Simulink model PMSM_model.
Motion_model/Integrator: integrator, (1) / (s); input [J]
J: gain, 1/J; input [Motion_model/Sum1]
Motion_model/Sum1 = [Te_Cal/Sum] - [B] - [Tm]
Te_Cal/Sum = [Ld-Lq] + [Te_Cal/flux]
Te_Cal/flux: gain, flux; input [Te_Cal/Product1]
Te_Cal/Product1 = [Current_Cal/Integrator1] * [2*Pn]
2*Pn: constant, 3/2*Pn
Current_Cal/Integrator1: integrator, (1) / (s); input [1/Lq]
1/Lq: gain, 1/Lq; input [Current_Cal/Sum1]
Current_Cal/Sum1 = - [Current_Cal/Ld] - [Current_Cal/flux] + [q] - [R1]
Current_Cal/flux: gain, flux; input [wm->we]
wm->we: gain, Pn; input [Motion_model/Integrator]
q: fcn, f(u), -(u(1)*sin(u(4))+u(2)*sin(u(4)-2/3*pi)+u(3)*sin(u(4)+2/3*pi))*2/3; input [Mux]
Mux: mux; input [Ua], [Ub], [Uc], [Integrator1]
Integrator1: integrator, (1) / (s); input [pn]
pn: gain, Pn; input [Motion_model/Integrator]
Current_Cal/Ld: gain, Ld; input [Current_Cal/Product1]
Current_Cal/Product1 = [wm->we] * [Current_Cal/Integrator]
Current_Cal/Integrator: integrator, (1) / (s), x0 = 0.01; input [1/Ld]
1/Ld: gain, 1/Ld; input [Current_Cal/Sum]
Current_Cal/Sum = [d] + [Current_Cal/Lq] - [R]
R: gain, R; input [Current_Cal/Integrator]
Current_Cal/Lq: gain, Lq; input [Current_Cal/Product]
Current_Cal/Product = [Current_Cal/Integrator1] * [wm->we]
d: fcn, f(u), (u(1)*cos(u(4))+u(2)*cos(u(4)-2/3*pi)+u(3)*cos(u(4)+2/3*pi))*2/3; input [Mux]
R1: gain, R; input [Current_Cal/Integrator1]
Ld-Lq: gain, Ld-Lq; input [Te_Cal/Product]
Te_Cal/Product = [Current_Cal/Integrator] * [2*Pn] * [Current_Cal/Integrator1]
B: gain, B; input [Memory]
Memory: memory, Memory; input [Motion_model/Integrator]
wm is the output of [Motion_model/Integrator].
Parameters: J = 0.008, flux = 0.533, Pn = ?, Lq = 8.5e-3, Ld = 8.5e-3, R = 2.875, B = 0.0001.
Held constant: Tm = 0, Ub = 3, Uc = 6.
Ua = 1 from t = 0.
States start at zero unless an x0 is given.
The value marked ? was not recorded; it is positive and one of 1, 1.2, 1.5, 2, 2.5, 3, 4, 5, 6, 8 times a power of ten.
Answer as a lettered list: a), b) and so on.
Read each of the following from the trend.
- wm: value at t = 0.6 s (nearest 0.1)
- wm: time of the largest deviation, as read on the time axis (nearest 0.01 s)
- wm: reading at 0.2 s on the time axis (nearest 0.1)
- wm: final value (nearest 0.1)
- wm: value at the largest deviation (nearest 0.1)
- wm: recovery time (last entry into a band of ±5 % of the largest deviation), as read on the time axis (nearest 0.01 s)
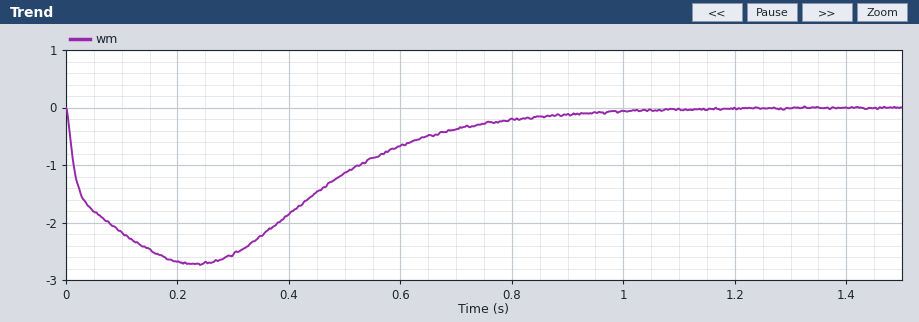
a) -0.7
b) 0.23 s
c) -2.7
d) 0.0
e) -2.7
f) 0.88 s
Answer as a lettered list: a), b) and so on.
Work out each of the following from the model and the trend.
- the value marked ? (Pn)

a) 2
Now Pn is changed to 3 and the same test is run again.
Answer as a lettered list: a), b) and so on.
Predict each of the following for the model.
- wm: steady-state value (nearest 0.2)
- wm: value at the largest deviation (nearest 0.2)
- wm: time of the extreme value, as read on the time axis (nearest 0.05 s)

a) 0.0
b) -1.8
c) 0.20 s
